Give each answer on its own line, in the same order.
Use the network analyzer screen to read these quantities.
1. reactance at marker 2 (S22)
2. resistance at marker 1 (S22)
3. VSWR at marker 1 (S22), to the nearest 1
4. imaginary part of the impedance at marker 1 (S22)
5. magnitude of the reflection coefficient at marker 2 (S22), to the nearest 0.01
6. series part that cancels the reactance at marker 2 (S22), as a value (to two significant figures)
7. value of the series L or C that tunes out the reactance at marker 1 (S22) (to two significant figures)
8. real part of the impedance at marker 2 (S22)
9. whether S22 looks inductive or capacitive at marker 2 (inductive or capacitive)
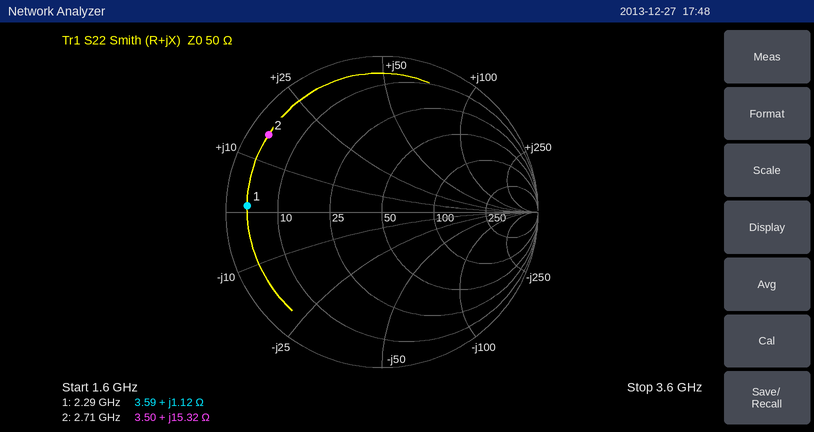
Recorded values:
+15.32 Ω
3.59 Ω
14
+1.12 Ω
0.88
3.8 pF
62 pF
3.50 Ω
inductive
